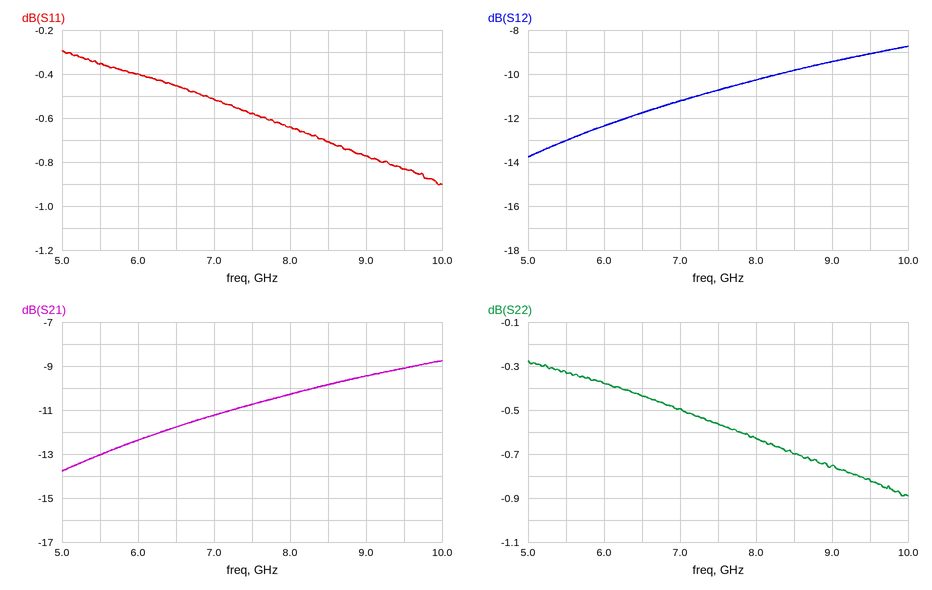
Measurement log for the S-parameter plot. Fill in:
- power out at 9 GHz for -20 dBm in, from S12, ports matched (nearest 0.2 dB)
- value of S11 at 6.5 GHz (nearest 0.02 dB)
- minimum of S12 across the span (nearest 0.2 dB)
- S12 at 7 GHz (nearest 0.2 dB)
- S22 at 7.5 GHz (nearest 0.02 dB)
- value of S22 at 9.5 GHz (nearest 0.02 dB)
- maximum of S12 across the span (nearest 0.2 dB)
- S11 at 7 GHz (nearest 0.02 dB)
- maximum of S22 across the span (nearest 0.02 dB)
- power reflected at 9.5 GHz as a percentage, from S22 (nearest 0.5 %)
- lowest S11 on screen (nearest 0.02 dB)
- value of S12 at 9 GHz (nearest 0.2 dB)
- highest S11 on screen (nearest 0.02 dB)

-29.4 dBm
-0.46 dB
-13.8 dB
-11.2 dB
-0.56 dB
-0.82 dB
-8.8 dB
-0.52 dB
-0.28 dB
83.0 %
-0.90 dB
-9.4 dB
-0.30 dB
